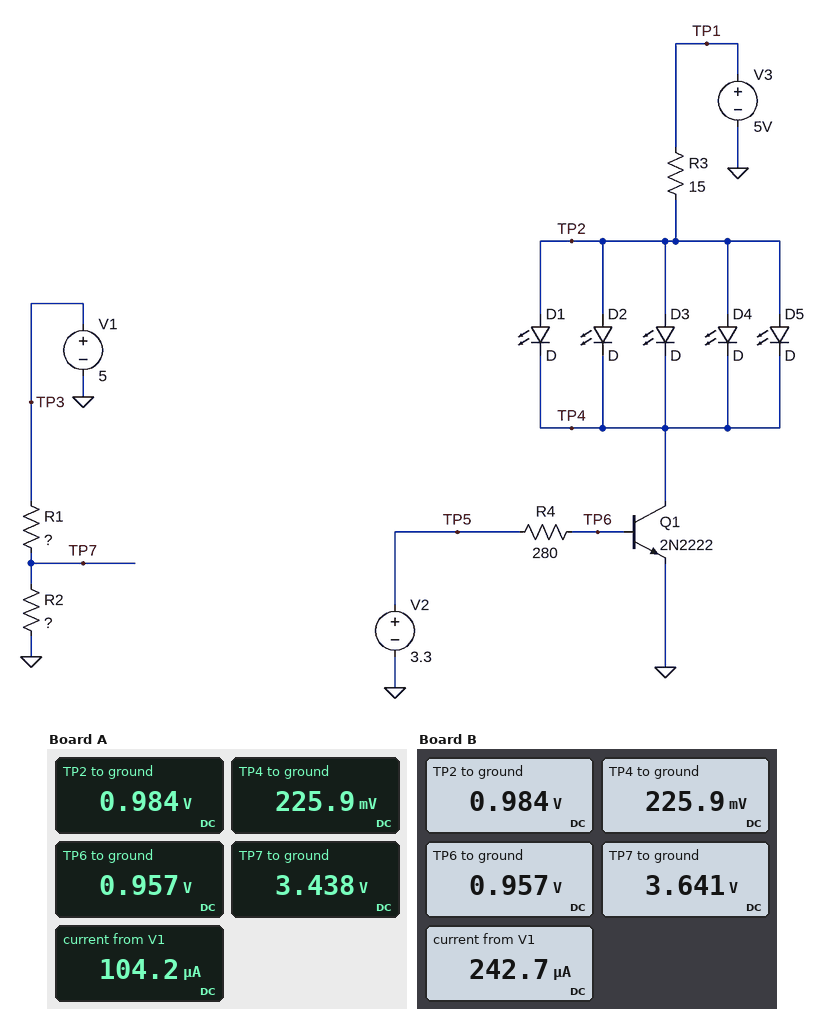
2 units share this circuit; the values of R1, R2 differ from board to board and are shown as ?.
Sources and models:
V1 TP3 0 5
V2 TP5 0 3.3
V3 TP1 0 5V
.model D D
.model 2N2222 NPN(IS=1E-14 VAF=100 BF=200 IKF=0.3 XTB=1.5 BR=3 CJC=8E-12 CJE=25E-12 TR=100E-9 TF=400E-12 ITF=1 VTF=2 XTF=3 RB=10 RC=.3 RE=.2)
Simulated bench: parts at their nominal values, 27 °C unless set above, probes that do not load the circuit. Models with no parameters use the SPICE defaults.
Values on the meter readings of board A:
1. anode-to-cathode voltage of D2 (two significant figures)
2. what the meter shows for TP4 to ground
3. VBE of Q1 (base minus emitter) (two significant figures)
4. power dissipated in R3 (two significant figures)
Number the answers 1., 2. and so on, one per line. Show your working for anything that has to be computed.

1. 984 mV - 225.9 mV = 760 mV
2. 225.9 mV
3. 957 mV = 960 mV
4. (5 V - 984 mV)^2 / 15 Ω = 1.1 W
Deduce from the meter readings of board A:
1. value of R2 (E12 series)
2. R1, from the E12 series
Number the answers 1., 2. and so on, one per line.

1. 33 kΩ
2. 15 kΩ
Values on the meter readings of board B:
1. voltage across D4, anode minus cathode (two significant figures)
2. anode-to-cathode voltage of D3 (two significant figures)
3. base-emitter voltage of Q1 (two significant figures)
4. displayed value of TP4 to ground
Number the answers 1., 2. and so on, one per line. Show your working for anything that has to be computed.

1. 984 mV - 225.9 mV = 760 mV
2. 984 mV - 225.9 mV = 760 mV
3. 957 mV = 960 mV
4. 225.9 mV
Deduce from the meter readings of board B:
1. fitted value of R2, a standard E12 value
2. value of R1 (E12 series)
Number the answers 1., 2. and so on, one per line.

1. 15 kΩ
2. 5.6 kΩ
